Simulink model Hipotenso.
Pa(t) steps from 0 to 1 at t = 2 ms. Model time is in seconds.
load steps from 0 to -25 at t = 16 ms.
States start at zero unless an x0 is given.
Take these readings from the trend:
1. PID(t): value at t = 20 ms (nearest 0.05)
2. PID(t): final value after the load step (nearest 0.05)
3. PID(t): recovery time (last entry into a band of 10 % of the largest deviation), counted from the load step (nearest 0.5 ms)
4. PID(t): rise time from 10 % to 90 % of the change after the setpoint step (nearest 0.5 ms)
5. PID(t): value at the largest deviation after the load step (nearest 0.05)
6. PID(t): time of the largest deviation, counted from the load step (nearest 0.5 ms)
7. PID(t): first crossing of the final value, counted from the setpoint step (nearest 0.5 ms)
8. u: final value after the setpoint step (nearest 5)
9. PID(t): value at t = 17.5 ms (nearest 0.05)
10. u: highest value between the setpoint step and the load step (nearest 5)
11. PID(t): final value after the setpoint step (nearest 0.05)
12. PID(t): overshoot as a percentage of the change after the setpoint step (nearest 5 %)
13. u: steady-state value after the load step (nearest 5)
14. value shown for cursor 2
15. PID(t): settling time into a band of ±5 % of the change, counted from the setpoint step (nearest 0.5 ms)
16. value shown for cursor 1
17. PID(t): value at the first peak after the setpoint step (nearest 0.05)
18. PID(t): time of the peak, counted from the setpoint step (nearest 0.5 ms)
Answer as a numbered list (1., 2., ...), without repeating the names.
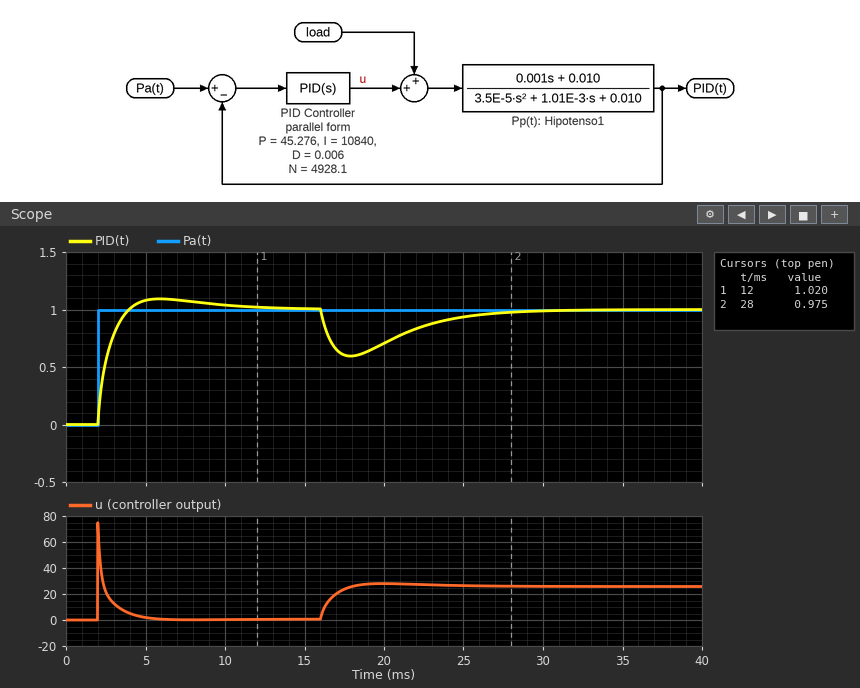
1. 0.70
2. 1.00
3. 10.5 ms
4. 1.5 ms
5. 0.60
6. 2.0 ms
7. 2.0 ms
8. 0
9. 0.60
10. 75
11. 1.00
12. 10 %
13. 25
14. 0.975
15. 7.0 ms
16. 1.020
17. 1.10
18. 4.0 ms
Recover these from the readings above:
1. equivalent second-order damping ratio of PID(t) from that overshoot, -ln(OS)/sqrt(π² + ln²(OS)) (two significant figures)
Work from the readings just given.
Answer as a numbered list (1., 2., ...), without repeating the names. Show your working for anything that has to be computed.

1. ln(0.1) = -2.303; 2.303 / sqrt(9.870 + 5.302) = 0.59
